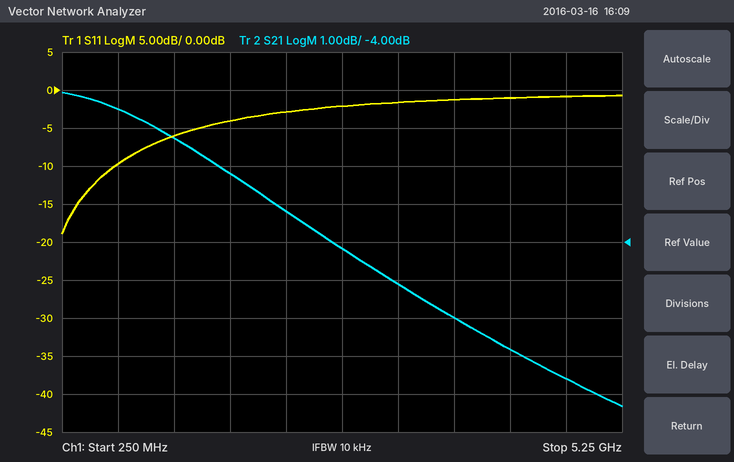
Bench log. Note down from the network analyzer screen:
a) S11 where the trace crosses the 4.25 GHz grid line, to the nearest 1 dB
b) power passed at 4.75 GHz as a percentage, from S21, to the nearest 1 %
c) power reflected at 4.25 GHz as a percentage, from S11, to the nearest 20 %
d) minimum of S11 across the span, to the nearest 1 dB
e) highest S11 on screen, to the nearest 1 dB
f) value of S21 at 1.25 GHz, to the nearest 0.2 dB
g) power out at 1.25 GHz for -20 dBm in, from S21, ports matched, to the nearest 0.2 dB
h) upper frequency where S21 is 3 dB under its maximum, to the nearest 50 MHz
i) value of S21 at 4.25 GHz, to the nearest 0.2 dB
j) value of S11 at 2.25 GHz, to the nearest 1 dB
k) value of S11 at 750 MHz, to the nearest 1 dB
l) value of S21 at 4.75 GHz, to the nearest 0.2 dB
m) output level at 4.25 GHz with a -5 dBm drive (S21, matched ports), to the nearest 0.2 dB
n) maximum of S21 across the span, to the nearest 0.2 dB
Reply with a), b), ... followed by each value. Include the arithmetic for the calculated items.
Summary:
a) -1 dB
b) 10^(-7.6/10) ≈ 17 %
c) 10^(-1/10) ≈ 79.4 %, so 80 % to the nearest 20 %
d) -19 dB
e) -1 dB
f) -1.2 dB
g) -20 dBm + (-1.2 dB) = -21.2 dBm
h) 2.20 GHz
i) -6.8 dB
j) -3 dB
k) -10 dB
l) -7.6 dB
m) -5 dBm + (-6.8 dB) = -11.8 dBm
n) 0.0 dB
